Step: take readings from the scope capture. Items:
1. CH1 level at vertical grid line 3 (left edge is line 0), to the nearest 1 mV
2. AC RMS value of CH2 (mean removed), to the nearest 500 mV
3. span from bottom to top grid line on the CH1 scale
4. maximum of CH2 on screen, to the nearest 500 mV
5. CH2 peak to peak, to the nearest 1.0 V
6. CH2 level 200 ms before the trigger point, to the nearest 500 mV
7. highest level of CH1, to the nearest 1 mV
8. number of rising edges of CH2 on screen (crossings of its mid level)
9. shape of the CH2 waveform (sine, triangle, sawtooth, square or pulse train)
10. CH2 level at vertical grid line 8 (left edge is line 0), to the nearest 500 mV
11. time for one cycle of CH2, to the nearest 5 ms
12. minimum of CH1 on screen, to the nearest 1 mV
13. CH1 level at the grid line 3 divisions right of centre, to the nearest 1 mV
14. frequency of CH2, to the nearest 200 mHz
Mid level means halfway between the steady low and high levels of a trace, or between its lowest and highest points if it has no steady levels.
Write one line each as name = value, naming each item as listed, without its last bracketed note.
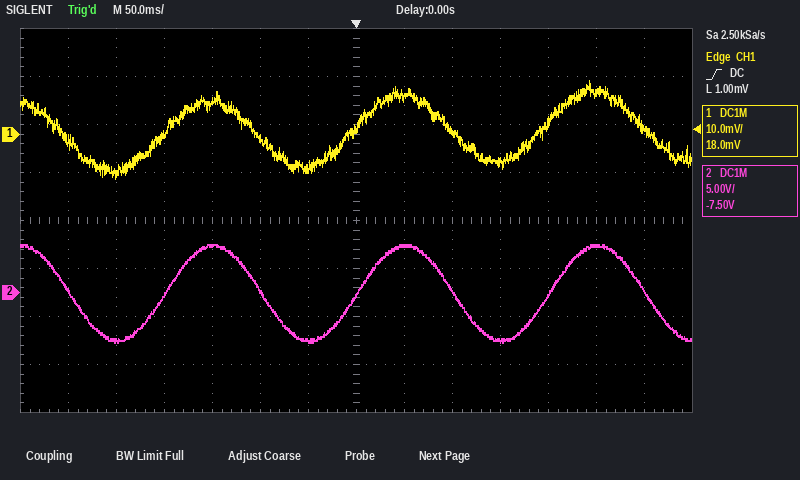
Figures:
CH1 level at vertical grid line 3 (left edge is line 0), to the nearest 1 mV = 0 mV
AC RMS value of CH2 (mean removed), to the nearest 500 mV = 3.5 V
span from bottom to top grid line on the CH1 scale = 80 mV
maximum of CH2 on screen, to the nearest 500 mV = 5.0 V
CH2 peak to peak, to the nearest 1.0 V = 10.0 V
CH2 level 200 ms before the trigger point, to the nearest 500 mV = -500 mV
highest level of CH1, to the nearest 1 mV = 11 mV
number of rising edges of CH2 on screen = 3
shape of the CH2 waveform = sine
CH2 level at vertical grid line 8 (left edge is line 0), to the nearest 500 mV = 5.0 V
time for one cycle of CH2, to the nearest 5 ms = 200 ms
minimum of CH1 on screen, to the nearest 1 mV = -9 mV
CH1 level at the grid line 3 divisions right of centre, to the nearest 1 mV = -6 mV
frequency of CH2, to the nearest 200 mHz = 5.0 Hz
